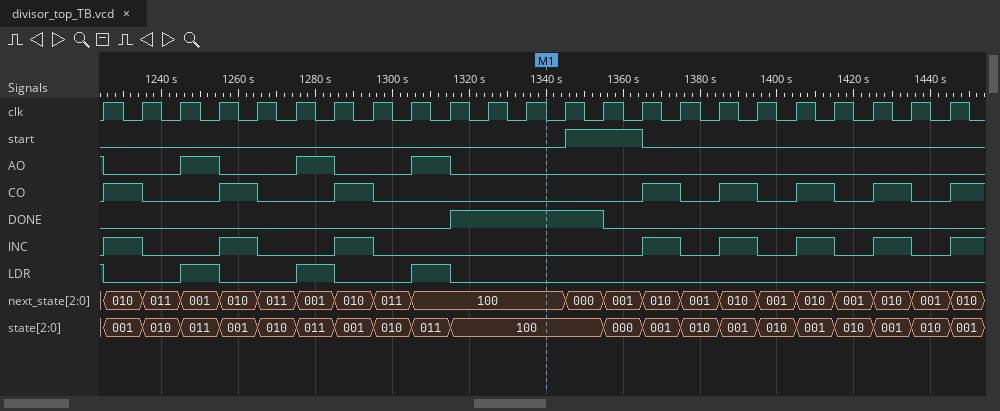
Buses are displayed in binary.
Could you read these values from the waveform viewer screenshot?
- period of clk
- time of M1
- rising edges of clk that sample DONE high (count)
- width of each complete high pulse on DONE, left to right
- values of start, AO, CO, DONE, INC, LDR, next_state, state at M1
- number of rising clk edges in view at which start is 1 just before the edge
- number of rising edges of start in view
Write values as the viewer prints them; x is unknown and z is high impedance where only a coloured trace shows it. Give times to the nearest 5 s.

10 s
1340 s
4
40 s
start=0, AO=0, CO=0, DONE=1, INC=0, LDR=0, next_state=100, state=100
2
1
